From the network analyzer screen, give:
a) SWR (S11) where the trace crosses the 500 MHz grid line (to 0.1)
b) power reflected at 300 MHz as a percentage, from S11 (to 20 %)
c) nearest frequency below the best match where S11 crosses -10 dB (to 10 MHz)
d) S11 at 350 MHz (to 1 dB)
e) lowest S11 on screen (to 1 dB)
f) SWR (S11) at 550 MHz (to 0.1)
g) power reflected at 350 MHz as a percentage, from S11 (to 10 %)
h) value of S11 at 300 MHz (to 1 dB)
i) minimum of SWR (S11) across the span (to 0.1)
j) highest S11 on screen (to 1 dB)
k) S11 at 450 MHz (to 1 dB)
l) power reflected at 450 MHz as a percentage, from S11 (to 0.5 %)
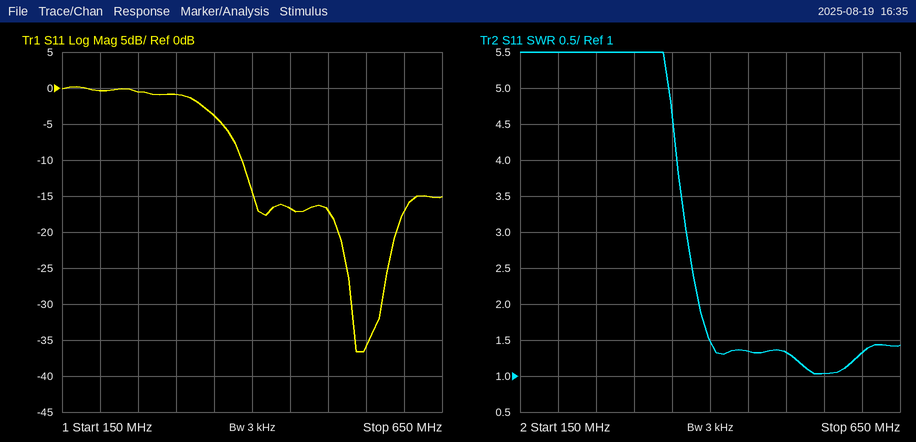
1.3
80 %
390 MHz
-4 dB
-37 dB
1.0
40 %
-1 dB
1.0
0 dB
-17 dB
2.0 %
